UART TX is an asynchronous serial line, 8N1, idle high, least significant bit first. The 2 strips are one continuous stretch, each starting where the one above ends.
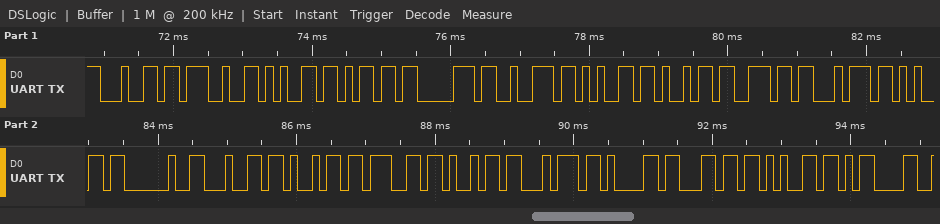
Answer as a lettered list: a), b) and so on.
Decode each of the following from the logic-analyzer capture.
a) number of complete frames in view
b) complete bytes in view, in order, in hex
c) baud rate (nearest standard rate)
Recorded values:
a) 21
b) 64 27 65 6D 70 72 65 69 6E 74 65 20 64 69 67 69 74 61 6C 65 0D
c) 9600 baud
